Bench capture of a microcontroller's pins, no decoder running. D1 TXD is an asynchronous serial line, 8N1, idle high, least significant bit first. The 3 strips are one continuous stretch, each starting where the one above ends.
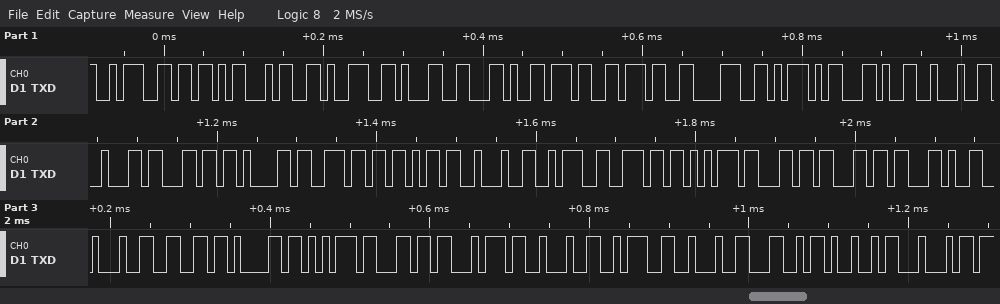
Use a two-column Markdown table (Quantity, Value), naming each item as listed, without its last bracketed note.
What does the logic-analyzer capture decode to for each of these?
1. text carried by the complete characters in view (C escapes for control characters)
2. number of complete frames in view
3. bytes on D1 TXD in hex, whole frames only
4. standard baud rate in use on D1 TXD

| Quantity | Value |
|---|---|
| text carried by the complete characters in view | ":[491,778],\"blank\":null,\"fault\":\"LID" |
| number of complete frames in view | 36 |
| bytes on D1 TXD in hex, whole frames only | 0x3A 0x5B 0x34 0x39 0x31 0x2C 0x37 0x37 0x38 0x5D 0x2C 0x22 0x62 0x6C 0x61 0x6E 0x6B 0x22 0x3A 0x6E 0x75 0x6C 0x6C 0x2C 0x22 0x66 0x61 0x75 0x6C 0x74 0x22 0x3A 0x22 0x4C 0x49 0x44 |
| standard baud rate in use on D1 TXD | 115200 baud |
